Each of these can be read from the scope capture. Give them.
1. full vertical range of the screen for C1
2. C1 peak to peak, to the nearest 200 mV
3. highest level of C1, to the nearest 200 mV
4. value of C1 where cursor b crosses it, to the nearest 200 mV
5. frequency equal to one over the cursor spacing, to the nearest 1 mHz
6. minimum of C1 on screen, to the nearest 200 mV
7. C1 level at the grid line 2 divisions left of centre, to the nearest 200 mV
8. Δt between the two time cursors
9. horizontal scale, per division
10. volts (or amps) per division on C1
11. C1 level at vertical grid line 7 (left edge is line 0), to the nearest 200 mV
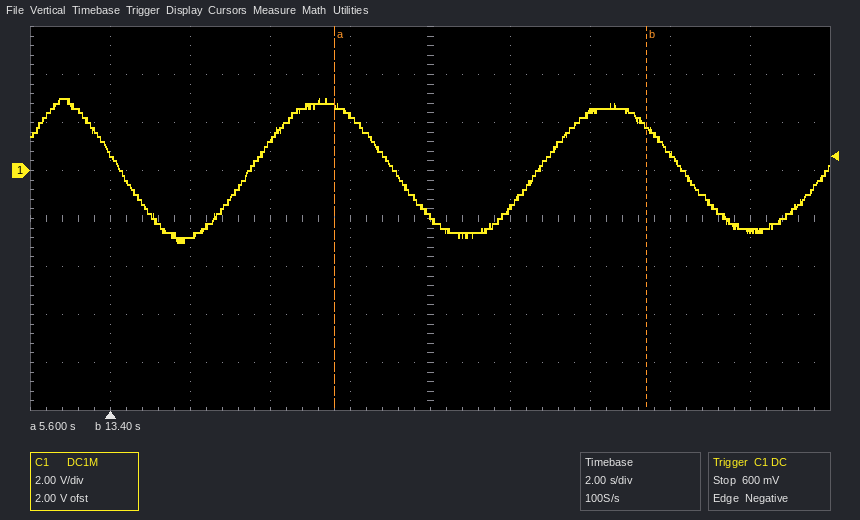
16 V
6.0 V
3.0 V
1.8 V
128 mHz
-3.0 V
1.2 V
7.8 s
2 s
2 V
2.4 V
